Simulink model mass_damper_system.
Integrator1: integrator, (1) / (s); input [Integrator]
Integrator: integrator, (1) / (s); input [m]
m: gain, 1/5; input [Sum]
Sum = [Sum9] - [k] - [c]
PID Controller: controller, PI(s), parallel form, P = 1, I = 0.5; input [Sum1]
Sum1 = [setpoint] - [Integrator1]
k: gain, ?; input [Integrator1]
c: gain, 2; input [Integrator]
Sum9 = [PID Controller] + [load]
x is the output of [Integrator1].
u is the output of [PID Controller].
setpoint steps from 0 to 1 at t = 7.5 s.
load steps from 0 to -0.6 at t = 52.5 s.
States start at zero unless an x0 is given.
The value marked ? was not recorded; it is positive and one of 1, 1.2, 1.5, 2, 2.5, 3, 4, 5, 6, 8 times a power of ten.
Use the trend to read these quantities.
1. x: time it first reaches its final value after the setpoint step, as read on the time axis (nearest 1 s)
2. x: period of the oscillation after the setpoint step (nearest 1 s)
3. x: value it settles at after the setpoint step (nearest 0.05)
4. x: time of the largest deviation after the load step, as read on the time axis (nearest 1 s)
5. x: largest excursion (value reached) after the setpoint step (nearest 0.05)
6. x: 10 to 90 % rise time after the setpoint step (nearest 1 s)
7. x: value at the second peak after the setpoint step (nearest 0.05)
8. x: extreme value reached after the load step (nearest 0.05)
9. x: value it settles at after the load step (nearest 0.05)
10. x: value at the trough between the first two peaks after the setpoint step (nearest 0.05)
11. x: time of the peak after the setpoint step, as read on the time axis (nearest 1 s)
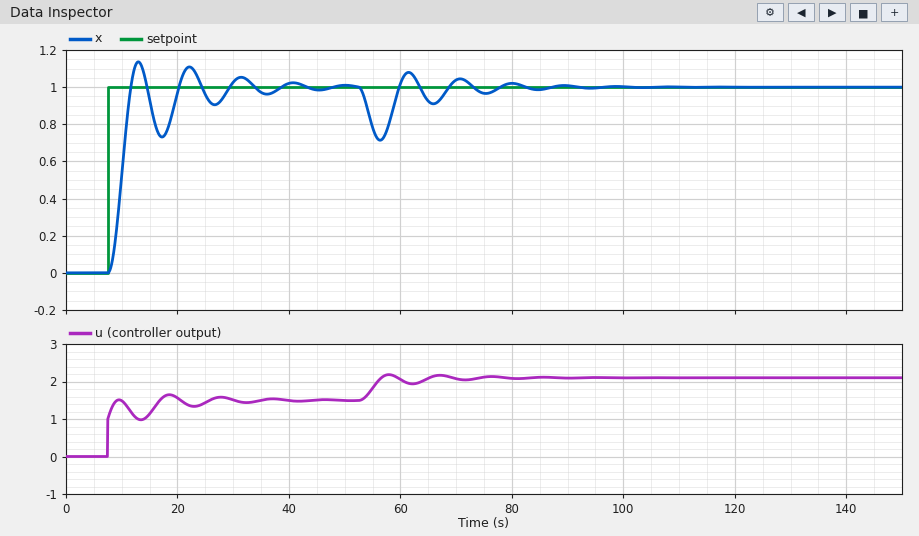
12 s
9 s
1.00
56 s
1.15
3 s
1.10
0.70
1.00
0.75
13 s
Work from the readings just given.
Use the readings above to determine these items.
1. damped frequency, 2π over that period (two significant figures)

0.70 rad/s
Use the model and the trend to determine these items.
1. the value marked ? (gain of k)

1.5
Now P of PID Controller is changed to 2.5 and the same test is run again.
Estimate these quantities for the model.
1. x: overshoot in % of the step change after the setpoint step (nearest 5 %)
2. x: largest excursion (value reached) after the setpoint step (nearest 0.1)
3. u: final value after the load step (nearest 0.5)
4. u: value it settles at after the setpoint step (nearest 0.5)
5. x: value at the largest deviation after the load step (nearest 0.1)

20 %
1.2
2.0
1.5
0.8
